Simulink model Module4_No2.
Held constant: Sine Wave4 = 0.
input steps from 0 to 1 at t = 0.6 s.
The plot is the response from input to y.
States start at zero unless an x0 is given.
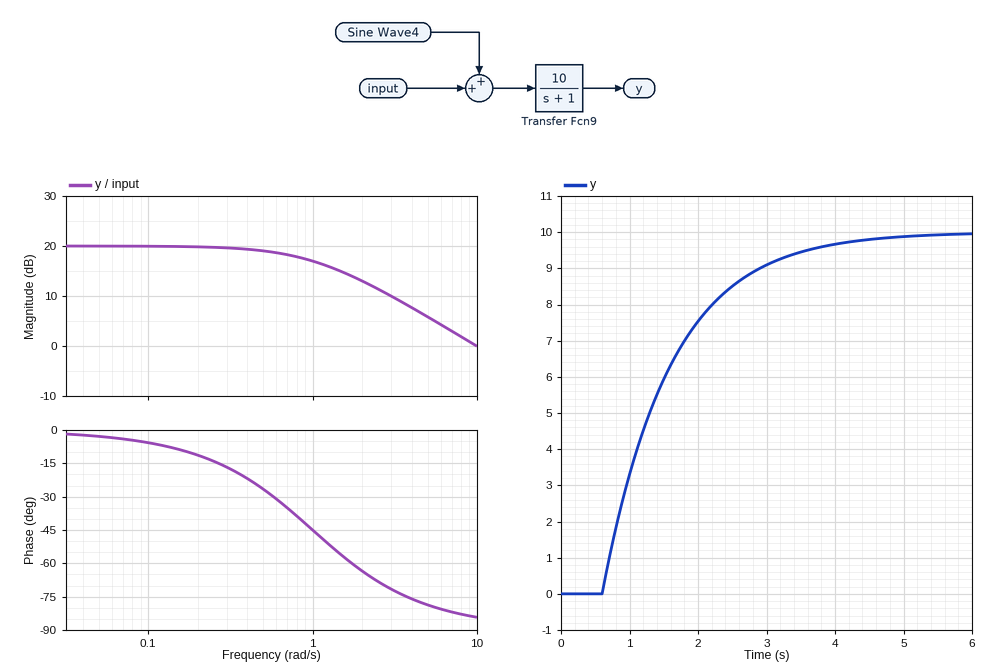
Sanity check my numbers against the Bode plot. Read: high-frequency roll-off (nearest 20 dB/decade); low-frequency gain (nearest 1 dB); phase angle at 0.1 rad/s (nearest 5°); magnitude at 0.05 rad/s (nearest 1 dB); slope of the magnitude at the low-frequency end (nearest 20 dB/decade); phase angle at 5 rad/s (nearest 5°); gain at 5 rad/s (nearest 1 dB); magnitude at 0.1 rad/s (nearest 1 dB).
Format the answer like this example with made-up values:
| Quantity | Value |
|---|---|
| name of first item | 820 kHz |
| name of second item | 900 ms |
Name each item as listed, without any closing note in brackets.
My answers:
| Quantity | Value |
|---|---|
| high-frequency roll-off | -20 dB/decade |
| low-frequency gain | 20 dB |
| phase angle at 0.1 rad/s | -5° |
| magnitude at 0.05 rad/s | 20 dB |
| slope of the magnitude at the low-frequency end | 0 dB/decade |
| phase angle at 5 rad/s | -80° |
| gain at 5 rad/s | 6 dB |
| magnitude at 0.1 rad/s | 20 dB |
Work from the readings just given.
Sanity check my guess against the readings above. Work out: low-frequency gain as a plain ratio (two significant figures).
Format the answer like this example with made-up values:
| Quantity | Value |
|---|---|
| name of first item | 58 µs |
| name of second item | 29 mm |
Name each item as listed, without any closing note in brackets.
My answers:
| Quantity | Value |
|---|---|
| low-frequency gain as a plain ratio | 10 |
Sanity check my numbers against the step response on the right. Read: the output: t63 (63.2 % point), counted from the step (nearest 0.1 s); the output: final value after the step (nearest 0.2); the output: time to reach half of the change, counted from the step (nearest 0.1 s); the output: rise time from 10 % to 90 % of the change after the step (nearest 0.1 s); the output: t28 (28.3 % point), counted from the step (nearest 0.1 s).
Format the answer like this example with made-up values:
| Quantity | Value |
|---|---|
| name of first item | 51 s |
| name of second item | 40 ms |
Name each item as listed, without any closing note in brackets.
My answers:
| Quantity | Value |
|---|---|
| the output: t63 (63.2 % point), counted from the step | 1.0 s |
| the output: final value after the step | 10.0 |
| the output: time to reach half of the change, counted from the step | 0.7 s |
| the output: rise time from 10 % to 90 % of the change after the step | 2.2 s |
| the output: t28 (28.3 % point), counted from the step | 0.3 s |
